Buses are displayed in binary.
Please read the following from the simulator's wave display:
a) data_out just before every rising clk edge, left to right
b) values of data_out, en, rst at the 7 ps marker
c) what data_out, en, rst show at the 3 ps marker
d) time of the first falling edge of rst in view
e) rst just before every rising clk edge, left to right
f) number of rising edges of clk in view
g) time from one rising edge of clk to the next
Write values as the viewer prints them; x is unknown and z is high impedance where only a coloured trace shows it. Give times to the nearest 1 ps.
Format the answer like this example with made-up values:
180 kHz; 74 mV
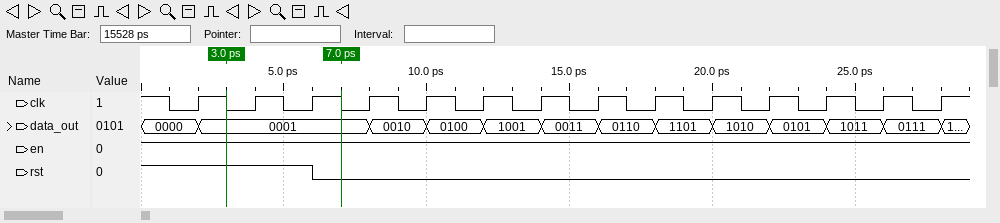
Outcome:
0000, 0001, 0001, 0001, 0010, 0100, 1001, 0011, 0110, 1101, 1010, 0101, 1011, 0111; data_out=0001, en=1, rst=0; data_out=0001, en=1, rst=1; 6 ps; 1 1 1 0 0 0 0 0 0 0 0 0 0 0; 14; 2 ps
